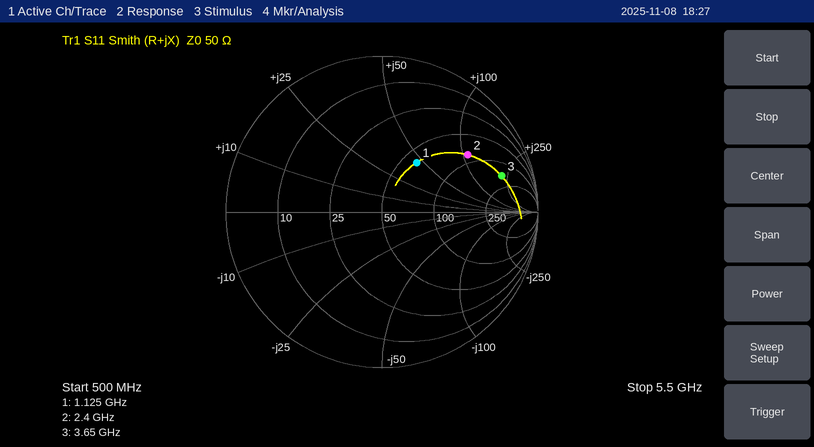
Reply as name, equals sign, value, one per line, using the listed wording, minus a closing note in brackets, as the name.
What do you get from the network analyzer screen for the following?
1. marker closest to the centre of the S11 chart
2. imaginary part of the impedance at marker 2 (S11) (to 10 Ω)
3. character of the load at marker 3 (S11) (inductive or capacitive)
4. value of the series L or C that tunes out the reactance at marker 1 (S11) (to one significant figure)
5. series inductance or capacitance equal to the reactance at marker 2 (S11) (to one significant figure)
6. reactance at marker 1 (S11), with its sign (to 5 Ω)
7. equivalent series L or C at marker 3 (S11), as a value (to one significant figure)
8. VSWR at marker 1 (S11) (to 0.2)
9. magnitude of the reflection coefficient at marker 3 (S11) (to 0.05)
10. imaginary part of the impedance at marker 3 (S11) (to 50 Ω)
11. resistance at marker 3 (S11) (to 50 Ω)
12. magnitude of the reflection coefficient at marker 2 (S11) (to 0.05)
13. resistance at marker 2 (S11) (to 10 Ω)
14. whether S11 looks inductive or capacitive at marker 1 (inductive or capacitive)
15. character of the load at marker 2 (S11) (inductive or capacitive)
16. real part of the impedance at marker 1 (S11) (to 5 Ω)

marker closest to the centre of the S11 chart = marker 1
imaginary part of the impedance at marker 2 (S11) = +110 Ω
character of the load at marker 3 (S11) = inductive
value of the series L or C that tunes out the reactance at marker 1 (S11) = 3 pF
series inductance or capacitance equal to the reactance at marker 2 (S11) = 7 nH
reactance at marker 1 (S11), with its sign = +45 Ω
equivalent series L or C at marker 3 (S11), as a value = 9 nH
VSWR at marker 1 (S11) = 2.2
magnitude of the reflection coefficient at marker 3 (S11) = 0.80
imaginary part of the impedance at marker 3 (S11) = +200 Ω
resistance at marker 3 (S11) = 150 Ω
magnitude of the reflection coefficient at marker 2 (S11) = 0.65
resistance at marker 2 (S11) = 80 Ω
whether S11 looks inductive or capacitive at marker 1 = inductive
character of the load at marker 2 (S11) = inductive
real part of the impedance at marker 1 (S11) = 60 Ω
